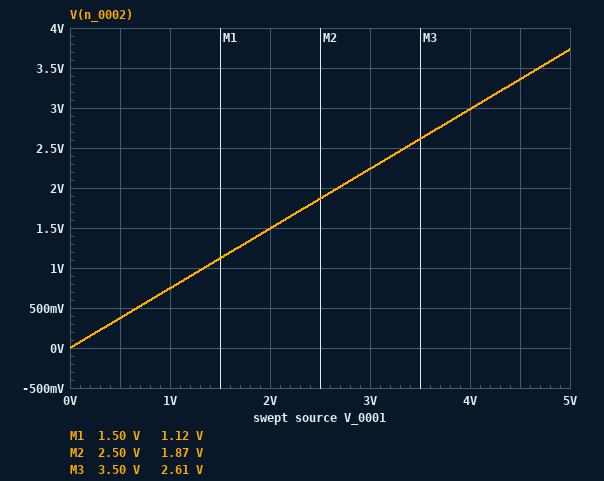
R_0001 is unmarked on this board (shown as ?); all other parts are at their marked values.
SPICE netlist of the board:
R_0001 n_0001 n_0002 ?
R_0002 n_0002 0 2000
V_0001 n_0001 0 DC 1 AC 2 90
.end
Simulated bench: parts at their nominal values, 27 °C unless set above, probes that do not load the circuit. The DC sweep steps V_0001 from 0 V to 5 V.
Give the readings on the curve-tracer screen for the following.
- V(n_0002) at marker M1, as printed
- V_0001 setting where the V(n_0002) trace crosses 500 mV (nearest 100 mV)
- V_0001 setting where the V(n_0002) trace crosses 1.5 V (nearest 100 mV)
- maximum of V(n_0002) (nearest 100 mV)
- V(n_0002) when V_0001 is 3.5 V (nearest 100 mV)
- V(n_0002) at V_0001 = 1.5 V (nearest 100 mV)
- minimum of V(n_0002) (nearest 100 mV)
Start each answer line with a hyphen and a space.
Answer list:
- 1.12 V
- 700 mV
- 2.0 V
- 3.7 V
- 2.6 V
- 1.1 V
- 0 V
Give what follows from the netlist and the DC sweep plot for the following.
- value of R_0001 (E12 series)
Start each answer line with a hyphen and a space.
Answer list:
- 680 Ω
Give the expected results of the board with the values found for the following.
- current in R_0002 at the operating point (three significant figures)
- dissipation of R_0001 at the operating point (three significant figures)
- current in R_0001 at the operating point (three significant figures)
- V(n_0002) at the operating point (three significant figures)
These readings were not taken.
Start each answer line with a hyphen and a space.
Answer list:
- 373 µA
- 94.7 µW
- 373 µA
- 746 mV
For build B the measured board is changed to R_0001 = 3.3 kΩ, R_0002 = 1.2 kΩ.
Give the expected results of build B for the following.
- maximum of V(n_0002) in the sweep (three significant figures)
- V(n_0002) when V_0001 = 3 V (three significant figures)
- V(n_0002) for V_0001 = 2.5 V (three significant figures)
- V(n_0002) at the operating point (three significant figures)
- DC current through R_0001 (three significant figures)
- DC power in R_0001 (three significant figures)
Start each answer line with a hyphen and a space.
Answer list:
- 1.33 V
- 800 mV
- 667 mV
- 267 mV
- 222 µA
- 163 µW
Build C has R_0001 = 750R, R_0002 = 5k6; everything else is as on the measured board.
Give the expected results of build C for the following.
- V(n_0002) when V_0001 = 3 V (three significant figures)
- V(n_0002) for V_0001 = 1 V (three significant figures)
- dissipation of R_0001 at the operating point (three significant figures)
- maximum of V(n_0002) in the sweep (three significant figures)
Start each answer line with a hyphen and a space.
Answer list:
- 2.65 V
- 882 mV
- 18.6 µW
- 4.41 V
